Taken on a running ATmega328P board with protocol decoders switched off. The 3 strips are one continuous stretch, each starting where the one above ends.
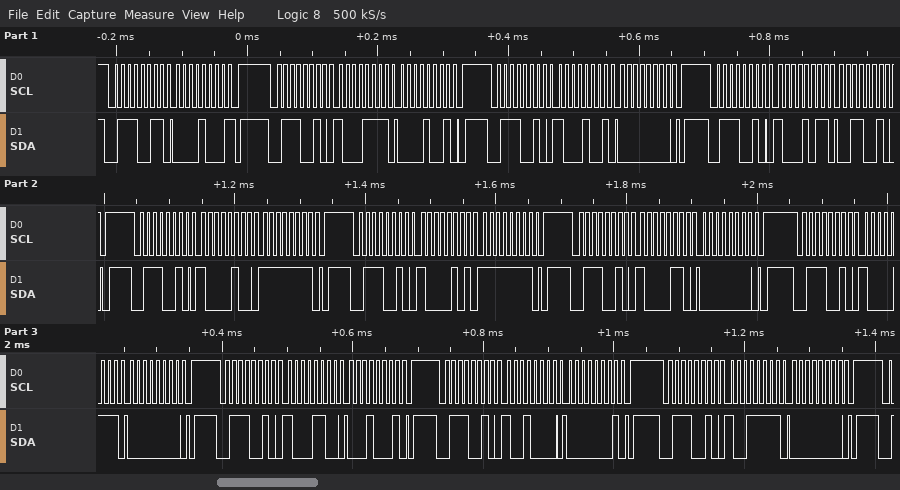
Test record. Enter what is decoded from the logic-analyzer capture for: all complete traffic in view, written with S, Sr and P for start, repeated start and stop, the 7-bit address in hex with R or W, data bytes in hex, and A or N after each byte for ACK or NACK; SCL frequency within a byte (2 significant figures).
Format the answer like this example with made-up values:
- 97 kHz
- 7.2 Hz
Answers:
- S 39R A 08 N P S 39W A 8F A 09 A P S 39W A 89 A 00 A P S 39W A 8B A 32 A P S 39W A 84 A FF A P S 39W A 85 A FF A P S 39W A 86 A 00 A P S 39W A 87 A 00 A P S 39W A 8C A 11 A P S 39W A 90 A 01 A P S 39W A 9F A 00 A P
- 100 kHz
